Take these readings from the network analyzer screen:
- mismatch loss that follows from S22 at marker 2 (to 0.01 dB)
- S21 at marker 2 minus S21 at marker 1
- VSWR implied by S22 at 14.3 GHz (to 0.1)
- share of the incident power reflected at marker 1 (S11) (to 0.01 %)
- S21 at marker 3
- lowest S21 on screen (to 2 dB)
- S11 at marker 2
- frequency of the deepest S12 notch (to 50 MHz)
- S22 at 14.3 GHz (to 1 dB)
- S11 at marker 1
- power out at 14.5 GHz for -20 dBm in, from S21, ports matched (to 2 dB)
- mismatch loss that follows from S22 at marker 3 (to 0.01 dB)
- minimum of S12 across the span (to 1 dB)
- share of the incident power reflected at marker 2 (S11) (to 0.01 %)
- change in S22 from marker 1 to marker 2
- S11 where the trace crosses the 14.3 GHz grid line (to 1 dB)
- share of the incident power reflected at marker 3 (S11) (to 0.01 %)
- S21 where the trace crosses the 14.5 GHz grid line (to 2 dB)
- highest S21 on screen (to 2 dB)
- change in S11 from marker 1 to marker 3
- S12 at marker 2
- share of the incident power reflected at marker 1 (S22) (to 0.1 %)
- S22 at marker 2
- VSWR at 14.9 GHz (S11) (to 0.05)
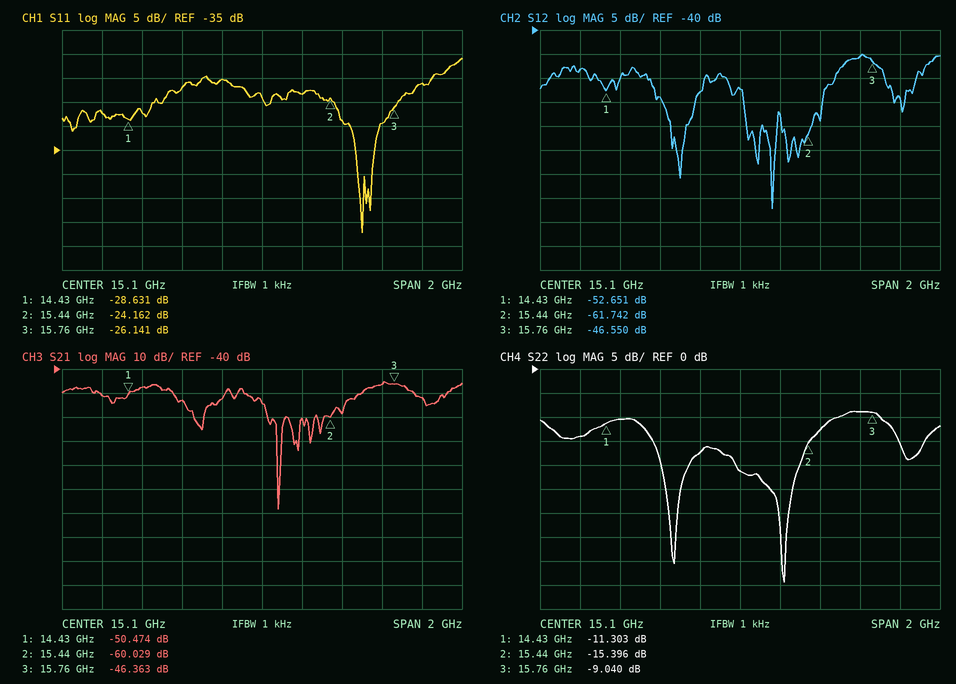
0.13 dB
-9.555 dB
1.5
0.14 %
-46.363 dB
-98 dB
-24.162 dB
15.25 GHz
-14 dB
-28.631 dB
-68 dBm
0.58 dB
-77 dB
0.38 %
-4.093 dB
-27 dB
0.24 %
-48 dB
-46 dB
2.490 dB
-61.742 dB
7.4 %
-15.396 dB
1.20
